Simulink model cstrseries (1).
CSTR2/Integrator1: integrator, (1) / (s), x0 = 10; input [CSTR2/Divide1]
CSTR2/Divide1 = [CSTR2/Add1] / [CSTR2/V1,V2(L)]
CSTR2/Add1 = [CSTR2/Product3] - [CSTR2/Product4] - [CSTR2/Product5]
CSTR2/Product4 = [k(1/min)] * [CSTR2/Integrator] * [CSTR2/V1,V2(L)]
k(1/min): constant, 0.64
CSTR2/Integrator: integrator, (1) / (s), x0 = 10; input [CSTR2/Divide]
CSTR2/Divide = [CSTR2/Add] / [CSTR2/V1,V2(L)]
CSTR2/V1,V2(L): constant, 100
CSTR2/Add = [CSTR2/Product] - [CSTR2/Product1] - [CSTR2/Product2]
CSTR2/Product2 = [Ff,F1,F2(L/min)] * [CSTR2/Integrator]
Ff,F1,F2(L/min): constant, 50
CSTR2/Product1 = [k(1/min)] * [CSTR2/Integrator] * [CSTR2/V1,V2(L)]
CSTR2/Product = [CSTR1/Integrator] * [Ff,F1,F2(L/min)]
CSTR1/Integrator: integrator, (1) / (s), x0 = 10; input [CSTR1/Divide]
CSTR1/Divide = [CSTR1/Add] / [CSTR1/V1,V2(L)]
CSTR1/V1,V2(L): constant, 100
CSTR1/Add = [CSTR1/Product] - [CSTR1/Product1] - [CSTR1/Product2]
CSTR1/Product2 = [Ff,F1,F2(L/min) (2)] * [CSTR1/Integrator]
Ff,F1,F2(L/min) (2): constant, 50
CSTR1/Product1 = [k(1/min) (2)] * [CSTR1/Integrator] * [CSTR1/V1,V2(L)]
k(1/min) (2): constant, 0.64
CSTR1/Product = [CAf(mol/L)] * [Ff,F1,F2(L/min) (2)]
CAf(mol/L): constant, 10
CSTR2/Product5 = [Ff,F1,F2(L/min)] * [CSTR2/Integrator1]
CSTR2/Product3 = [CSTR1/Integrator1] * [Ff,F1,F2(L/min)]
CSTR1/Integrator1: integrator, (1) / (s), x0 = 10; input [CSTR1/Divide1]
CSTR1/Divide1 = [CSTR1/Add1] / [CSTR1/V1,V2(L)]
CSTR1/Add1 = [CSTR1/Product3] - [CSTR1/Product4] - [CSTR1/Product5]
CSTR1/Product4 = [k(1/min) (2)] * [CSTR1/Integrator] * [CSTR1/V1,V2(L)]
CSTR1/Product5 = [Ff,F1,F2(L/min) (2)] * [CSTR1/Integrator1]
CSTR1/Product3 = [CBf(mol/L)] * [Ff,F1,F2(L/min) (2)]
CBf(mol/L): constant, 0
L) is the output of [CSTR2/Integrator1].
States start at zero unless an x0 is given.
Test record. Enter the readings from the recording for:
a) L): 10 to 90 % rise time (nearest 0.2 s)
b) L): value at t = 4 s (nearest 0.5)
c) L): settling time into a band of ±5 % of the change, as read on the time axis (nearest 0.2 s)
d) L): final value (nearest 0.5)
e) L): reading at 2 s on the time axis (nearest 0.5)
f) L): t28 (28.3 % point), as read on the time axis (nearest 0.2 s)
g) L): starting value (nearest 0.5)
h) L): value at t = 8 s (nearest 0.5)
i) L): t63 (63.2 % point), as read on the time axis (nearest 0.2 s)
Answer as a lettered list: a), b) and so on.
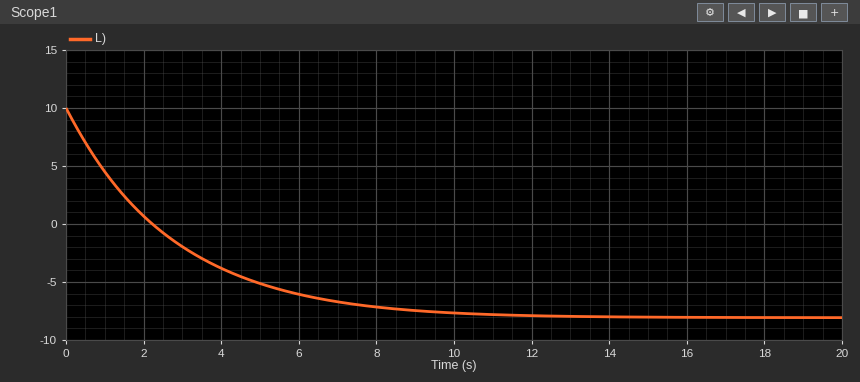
a) 6.0 s
b) -4.0
c) 8.0 s
d) -8.0
e) 0.5
f) 1.0 s
g) 10.0
h) -7.0
i) 2.8 s
